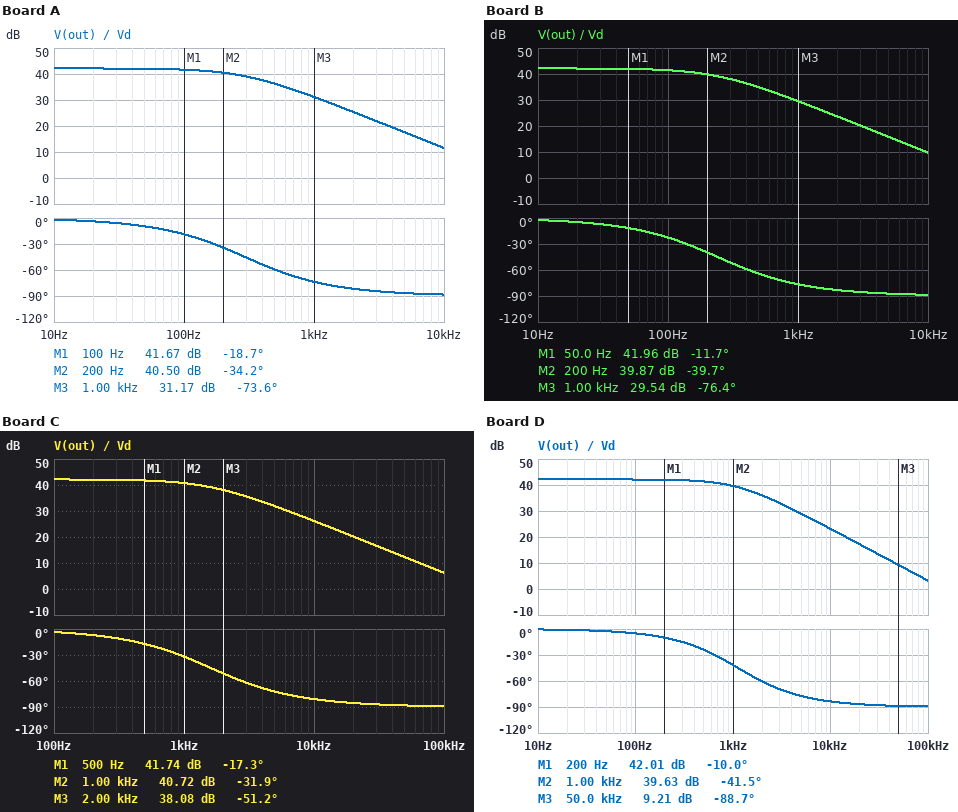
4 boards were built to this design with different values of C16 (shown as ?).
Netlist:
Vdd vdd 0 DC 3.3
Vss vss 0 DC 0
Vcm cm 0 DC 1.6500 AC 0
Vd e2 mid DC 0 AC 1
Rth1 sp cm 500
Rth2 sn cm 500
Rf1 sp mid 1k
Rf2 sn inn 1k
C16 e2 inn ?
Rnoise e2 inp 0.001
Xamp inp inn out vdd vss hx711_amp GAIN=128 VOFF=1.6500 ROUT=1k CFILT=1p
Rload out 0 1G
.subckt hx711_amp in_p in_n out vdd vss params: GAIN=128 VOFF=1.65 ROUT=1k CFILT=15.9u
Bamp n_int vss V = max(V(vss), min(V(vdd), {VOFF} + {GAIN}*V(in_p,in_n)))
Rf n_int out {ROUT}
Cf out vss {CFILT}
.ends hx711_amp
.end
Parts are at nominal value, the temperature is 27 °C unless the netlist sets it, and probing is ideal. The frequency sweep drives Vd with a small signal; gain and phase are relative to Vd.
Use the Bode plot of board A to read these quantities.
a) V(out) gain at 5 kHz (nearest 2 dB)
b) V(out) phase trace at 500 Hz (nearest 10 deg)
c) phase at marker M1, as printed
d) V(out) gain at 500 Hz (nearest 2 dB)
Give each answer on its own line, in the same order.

18 dB
-60 deg
-18.7 deg
36 dB
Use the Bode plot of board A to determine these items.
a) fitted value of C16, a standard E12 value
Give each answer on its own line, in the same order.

180 nF
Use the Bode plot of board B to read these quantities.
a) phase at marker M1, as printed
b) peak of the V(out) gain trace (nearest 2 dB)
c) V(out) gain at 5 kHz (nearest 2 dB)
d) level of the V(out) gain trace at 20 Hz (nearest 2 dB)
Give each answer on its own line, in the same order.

-11.7 deg
42 dB
16 dB
42 dB
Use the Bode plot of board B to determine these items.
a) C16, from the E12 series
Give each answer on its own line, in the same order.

220 nF
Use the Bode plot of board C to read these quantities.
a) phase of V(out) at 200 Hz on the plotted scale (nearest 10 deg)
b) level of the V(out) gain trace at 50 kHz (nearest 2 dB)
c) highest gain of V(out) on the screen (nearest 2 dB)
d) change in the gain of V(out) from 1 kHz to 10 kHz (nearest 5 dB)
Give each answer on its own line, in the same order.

-10 deg
12 dB
42 dB
-15 dB
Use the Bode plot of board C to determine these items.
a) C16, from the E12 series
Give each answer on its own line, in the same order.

33 nF
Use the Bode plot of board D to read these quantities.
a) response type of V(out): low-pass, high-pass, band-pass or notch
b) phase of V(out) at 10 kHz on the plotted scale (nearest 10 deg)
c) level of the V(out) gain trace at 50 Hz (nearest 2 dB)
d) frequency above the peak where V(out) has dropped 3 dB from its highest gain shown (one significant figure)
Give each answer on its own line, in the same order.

low-pass
-80 deg
42 dB
1 kHz
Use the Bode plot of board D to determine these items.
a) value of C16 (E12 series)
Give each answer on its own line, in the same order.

47 nF
